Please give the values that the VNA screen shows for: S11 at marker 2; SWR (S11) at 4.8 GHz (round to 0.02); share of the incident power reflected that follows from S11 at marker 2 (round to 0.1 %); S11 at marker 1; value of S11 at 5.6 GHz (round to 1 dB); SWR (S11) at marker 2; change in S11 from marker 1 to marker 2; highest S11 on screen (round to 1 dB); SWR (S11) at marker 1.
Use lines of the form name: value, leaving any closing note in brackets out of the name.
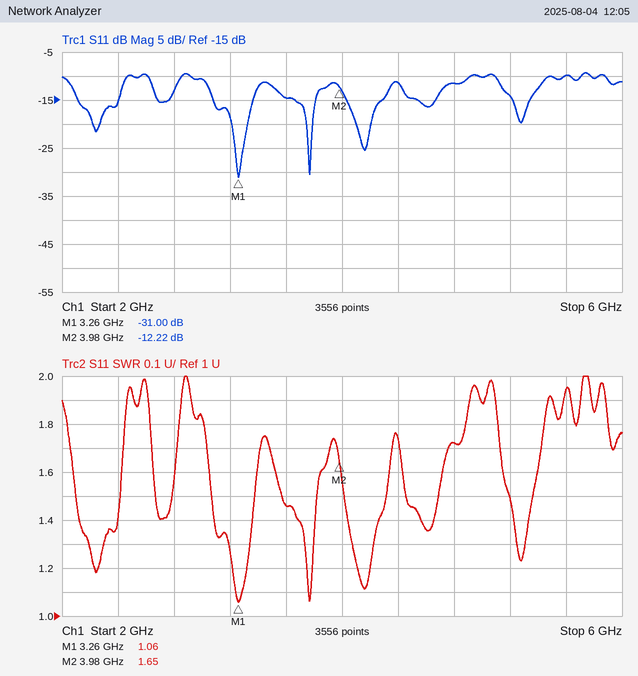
S11 at marker 2: -12.22 dB
SWR (S11) at 4.8 GHz: 1.72
share of the incident power reflected that follows from S11 at marker 2: 6.0 %
S11 at marker 1: -31.00 dB
value of S11 at 5.6 GHz: -10 dB
SWR (S11) at marker 2: 1.65
change in S11 from marker 1 to marker 2: 18.78 dB
highest S11 on screen: -9 dB
SWR (S11) at marker 1: 1.06
